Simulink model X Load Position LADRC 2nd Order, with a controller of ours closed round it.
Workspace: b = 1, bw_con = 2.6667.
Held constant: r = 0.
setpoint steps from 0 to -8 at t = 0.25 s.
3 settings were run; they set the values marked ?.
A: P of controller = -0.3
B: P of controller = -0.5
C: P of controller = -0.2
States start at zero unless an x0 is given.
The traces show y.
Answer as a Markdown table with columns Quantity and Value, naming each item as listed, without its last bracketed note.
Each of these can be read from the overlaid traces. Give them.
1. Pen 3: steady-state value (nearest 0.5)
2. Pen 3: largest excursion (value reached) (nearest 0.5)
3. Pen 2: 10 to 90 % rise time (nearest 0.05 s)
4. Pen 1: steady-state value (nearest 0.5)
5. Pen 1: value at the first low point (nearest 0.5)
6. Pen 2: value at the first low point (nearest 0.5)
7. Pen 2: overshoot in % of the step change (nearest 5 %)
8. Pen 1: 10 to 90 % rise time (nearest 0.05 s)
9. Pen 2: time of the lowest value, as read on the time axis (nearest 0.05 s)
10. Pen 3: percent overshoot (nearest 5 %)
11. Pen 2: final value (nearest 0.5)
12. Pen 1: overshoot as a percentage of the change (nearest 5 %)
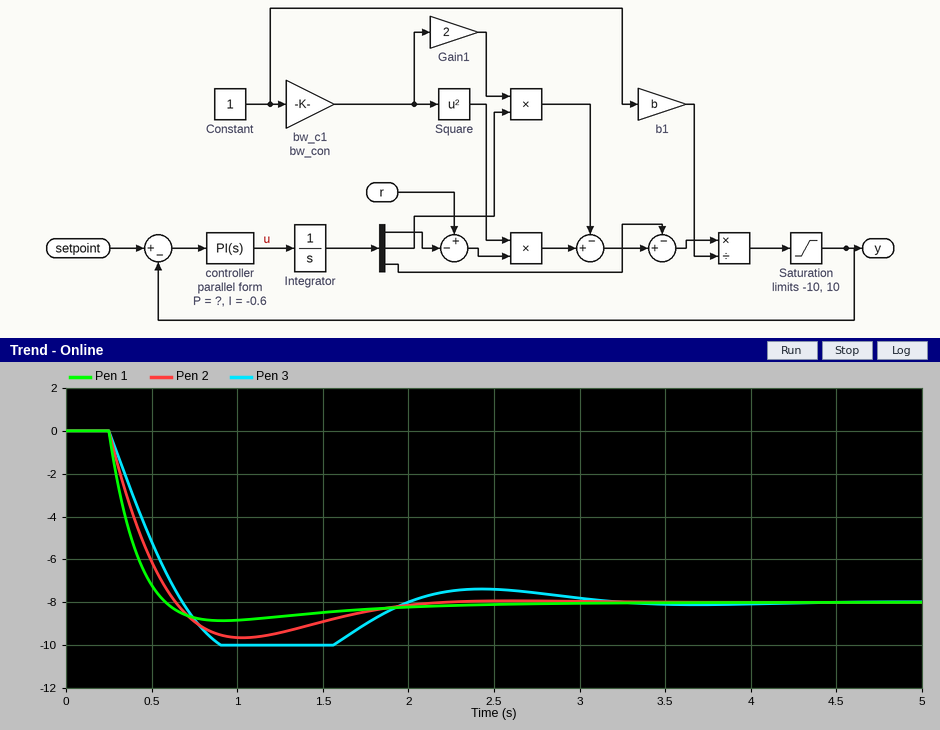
| Quantity | Value |
|---|---|
| Pen 3: steady-state value | -8.0 |
| Pen 3: largest excursion (value reached) | -10.0 |
| Pen 2: 10 to 90 % rise time | 0.30 s |
| Pen 1: steady-state value | -8.0 |
| Pen 1: value at the first low point | -9.0 |
| Pen 2: value at the first low point | -9.5 |
| Pen 2: overshoot in % of the step change | 20 % |
| Pen 1: 10 to 90 % rise time | 0.25 s |
| Pen 2: time of the lowest value, as read on the time axis | 1.05 s |
| Pen 3: percent overshoot | 25 % |
| Pen 2: final value | -8.0 |
| Pen 1: overshoot as a percentage of the change | 10 % |
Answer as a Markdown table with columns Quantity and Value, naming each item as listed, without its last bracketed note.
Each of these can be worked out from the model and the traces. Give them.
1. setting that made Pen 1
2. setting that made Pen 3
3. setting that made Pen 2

| Quantity | Value |
|---|---|
| setting that made Pen 1 | B |
| setting that made Pen 3 | C |
| setting that made Pen 2 | A |
